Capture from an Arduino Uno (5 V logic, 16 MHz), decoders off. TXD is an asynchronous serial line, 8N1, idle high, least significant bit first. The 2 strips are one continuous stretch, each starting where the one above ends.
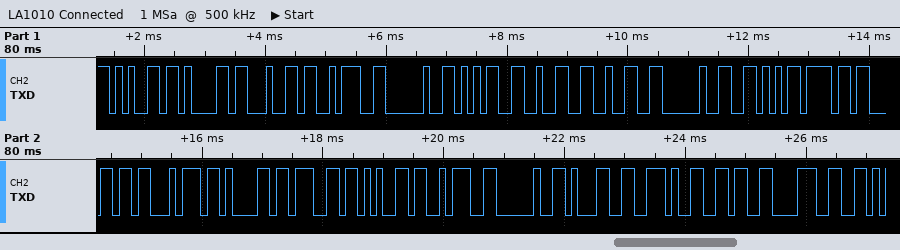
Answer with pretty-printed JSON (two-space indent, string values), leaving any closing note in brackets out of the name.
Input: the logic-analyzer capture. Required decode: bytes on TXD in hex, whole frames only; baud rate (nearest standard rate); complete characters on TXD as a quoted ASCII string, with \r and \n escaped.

{
  "bytes on TXD in hex, whole frames only": "65 61 64 3A 20 35 32 32 20 56 6F 6C 74 61 67 65 3A 20 31 2E 36 38",
  "baud rate": "9600 baud",
  "complete characters on TXD as a quoted ASCII string, with \\r and \\n escaped": "\"ead: 522 Voltage: 1.68\""
}
